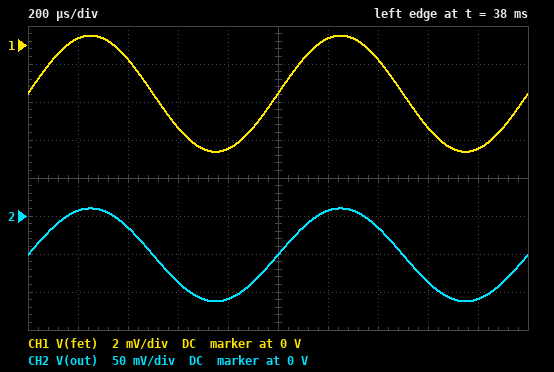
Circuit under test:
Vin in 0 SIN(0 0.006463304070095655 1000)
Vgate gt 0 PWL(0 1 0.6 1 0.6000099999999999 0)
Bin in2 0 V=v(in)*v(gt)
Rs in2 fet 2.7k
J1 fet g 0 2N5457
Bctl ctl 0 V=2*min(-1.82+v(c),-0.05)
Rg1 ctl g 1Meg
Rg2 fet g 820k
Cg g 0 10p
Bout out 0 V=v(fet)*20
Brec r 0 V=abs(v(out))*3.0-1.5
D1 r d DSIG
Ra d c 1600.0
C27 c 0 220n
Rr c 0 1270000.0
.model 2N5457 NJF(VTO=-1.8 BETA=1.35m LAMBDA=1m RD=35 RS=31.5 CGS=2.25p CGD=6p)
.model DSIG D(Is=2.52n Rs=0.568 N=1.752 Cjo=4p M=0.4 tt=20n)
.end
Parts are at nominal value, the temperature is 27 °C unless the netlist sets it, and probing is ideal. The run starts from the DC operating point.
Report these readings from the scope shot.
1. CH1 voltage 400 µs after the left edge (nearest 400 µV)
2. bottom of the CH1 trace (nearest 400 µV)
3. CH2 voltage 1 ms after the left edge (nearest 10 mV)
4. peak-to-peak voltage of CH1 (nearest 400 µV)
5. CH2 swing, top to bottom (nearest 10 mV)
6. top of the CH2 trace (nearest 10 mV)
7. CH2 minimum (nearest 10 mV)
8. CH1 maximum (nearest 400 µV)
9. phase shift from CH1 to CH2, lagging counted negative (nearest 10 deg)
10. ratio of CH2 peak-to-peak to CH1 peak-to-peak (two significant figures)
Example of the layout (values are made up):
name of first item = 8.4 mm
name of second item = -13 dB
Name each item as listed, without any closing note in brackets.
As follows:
CH1 voltage 400 µs after the left edge = -800 µV
bottom of the CH1 trace = -5.6 mV
CH2 voltage 1 ms after the left edge = -50 mV
peak-to-peak voltage of CH1 = 6.0 mV
CH2 swing, top to bottom = 120 mV
top of the CH2 trace = 10 mV
CH2 minimum = -110 mV
CH1 maximum = 400 µV
phase shift from CH1 to CH2, lagging counted negative = 0 deg
ratio of CH2 peak-to-peak to CH1 peak-to-peak = 20
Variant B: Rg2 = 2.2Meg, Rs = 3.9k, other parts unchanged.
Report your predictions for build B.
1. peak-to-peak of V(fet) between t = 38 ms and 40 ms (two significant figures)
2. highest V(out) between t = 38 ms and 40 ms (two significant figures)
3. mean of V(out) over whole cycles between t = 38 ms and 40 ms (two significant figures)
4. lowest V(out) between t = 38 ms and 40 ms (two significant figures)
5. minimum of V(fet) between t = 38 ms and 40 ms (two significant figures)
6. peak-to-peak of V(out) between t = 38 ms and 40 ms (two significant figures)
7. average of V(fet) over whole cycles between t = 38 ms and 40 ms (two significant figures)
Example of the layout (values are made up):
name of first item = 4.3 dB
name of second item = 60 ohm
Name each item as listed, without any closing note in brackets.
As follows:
peak-to-peak of V(fet) between t = 38 ms and 40 ms = 13 mV
highest V(out) between t = 38 ms and 40 ms = 40 mV
mean of V(out) over whole cycles between t = 38 ms and 40 ms = -89 mV
lowest V(out) between t = 38 ms and 40 ms = -220 mV
minimum of V(fet) between t = 38 ms and 40 ms = -11 mV
peak-to-peak of V(out) between t = 38 ms and 40 ms = 260 mV
average of V(fet) over whole cycles between t = 38 ms and 40 ms = -4.4 mV
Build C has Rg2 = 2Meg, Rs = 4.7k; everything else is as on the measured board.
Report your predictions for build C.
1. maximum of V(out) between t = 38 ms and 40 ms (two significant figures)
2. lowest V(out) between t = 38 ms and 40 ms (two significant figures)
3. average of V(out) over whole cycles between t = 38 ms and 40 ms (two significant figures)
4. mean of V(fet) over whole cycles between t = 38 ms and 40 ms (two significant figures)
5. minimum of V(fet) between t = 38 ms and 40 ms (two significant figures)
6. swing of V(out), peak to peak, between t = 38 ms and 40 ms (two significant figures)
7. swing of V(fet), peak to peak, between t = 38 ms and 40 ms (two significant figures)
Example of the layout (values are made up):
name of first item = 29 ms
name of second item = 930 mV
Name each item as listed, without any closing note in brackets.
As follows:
maximum of V(out) between t = 38 ms and 40 ms = 15 mV
lowest V(out) between t = 38 ms and 40 ms = -240 mV
average of V(out) over whole cycles between t = 38 ms and 40 ms = -110 mV
mean of V(fet) over whole cycles between t = 38 ms and 40 ms = -5.7 mV
minimum of V(fet) between t = 38 ms and 40 ms = -12 mV
swing of V(out), peak to peak, between t = 38 ms and 40 ms = 260 mV
swing of V(fet), peak to peak, between t = 38 ms and 40 ms = 13 mV
